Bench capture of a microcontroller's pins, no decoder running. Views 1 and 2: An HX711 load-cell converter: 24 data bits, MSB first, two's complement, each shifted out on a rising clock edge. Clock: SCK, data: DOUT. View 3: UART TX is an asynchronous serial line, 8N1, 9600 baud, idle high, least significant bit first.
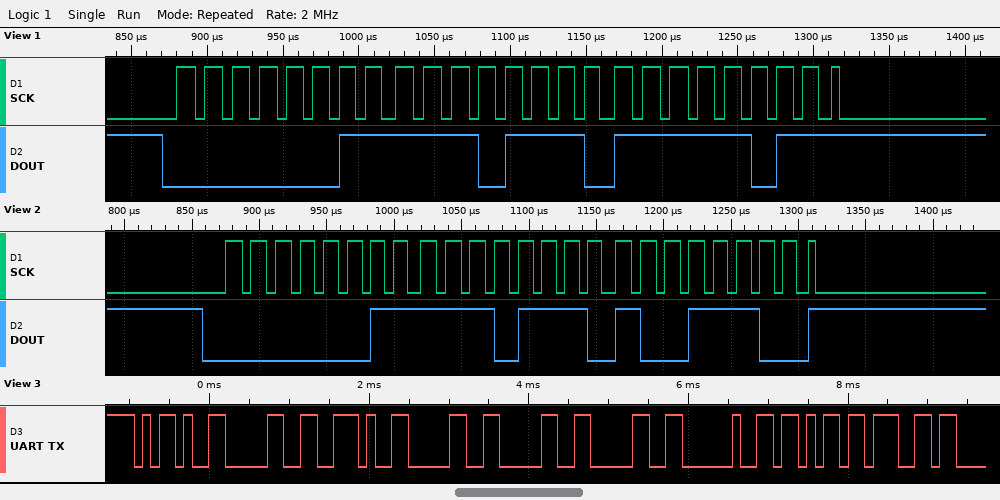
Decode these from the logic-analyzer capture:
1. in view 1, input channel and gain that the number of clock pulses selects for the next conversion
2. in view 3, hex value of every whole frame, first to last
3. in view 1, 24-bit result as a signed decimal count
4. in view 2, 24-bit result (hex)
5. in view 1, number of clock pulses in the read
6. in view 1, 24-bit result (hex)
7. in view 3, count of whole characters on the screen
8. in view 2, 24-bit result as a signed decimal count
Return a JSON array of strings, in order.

["channel A, gain 128", "2D 30 2E 30 30 30 20 6B 67", "257787", "0x03EE9C", "25", "0x03EEFB", "9", "257692"]
